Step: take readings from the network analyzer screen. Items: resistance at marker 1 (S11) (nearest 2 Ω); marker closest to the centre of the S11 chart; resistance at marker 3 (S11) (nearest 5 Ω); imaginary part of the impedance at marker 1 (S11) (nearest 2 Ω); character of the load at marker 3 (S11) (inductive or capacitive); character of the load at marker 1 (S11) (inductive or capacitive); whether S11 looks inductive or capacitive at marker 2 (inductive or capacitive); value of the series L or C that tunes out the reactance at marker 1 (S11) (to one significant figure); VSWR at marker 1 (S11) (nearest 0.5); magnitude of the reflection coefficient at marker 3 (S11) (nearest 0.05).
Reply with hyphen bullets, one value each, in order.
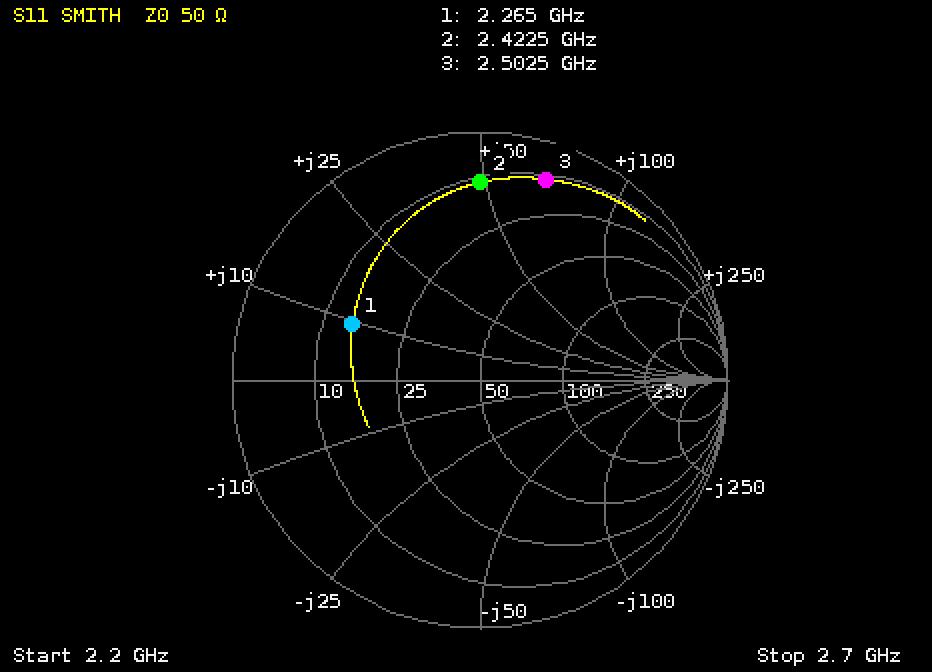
- 14 Ω
- marker 1
- 10 Ω
- +10 Ω
- inductive
- inductive
- inductive
- 7 pF
- 3.5
- 0.85
